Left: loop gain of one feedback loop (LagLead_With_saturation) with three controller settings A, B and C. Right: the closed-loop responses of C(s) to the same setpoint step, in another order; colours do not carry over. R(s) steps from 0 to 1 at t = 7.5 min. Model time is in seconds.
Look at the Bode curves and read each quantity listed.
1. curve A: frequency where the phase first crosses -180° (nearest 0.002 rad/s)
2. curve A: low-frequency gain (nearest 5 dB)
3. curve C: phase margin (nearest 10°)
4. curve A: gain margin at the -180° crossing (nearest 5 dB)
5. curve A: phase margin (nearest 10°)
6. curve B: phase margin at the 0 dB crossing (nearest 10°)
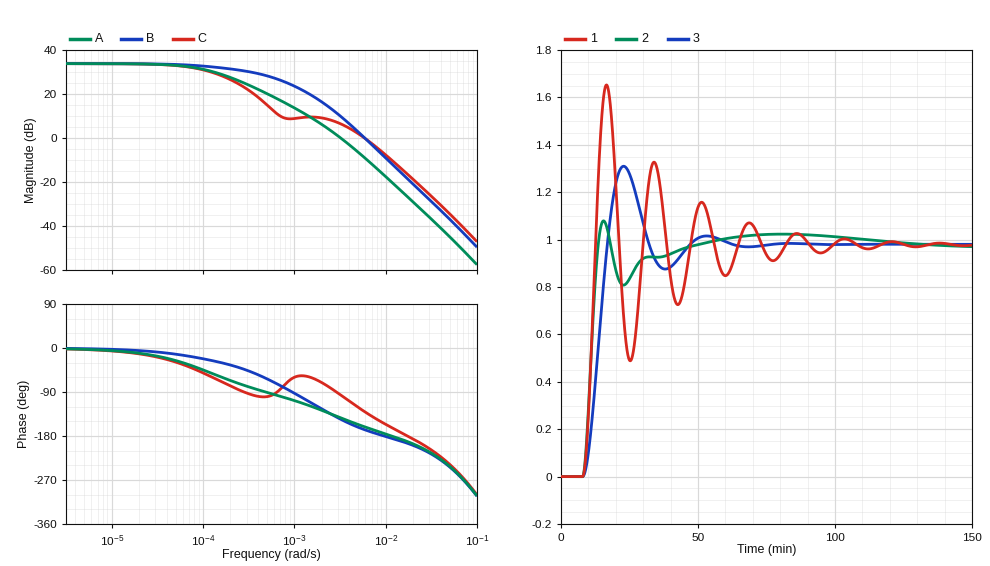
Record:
0.012 rad/s
35 dB
50°
20 dB
40°
10°
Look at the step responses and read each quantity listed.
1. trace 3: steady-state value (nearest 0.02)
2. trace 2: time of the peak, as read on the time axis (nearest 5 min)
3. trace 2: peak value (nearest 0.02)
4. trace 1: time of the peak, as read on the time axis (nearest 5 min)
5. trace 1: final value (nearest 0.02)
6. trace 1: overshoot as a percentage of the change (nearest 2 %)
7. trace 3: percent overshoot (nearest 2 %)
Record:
0.98
15 min
1.08
15 min
0.98
68 %
34 %
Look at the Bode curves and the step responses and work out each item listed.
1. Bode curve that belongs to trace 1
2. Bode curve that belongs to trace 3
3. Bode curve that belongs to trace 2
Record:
B
A
C
